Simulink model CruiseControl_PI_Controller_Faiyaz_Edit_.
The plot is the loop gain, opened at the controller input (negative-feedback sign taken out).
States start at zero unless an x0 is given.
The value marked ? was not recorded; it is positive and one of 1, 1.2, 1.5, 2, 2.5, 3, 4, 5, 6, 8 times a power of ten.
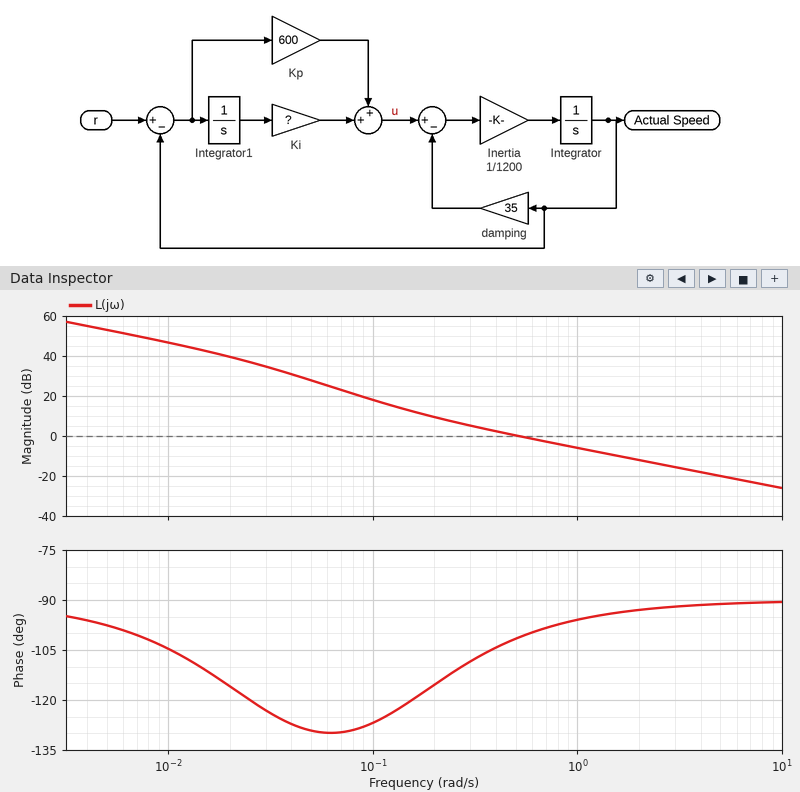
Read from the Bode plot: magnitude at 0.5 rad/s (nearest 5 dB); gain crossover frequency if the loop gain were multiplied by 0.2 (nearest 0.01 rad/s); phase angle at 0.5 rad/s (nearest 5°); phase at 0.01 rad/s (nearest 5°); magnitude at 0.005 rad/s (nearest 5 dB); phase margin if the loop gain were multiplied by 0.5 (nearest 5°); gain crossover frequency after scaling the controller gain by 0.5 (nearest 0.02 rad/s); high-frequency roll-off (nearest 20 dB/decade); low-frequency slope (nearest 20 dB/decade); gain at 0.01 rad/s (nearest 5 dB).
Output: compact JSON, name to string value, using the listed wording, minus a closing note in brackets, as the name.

{"magnitude at 0.5 rad/s": "0 dB", "gain crossover frequency if the loop gain were multiplied by 0.2": "0.14 rad/s", "phase angle at 0.5 rad/s": "-100°", "phase at 0.01 rad/s": "-105°", "magnitude at 0.005 rad/s": "55 dB", "phase margin if the loop gain were multiplied by 0.5": "70°", "gain crossover frequency after scaling the controller gain by 0.5": "0.28 rad/s", "high-frequency roll-off": "-20 dB/decade", "low-frequency slope": "-20 dB/decade", "gain at 0.01 rad/s": "45 dB"}
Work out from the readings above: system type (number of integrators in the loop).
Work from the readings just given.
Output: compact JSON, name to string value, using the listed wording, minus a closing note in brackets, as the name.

{"system type": "1"}
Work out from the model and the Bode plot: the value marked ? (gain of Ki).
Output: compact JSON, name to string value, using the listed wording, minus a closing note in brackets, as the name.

{"the value marked ?": "80"}
